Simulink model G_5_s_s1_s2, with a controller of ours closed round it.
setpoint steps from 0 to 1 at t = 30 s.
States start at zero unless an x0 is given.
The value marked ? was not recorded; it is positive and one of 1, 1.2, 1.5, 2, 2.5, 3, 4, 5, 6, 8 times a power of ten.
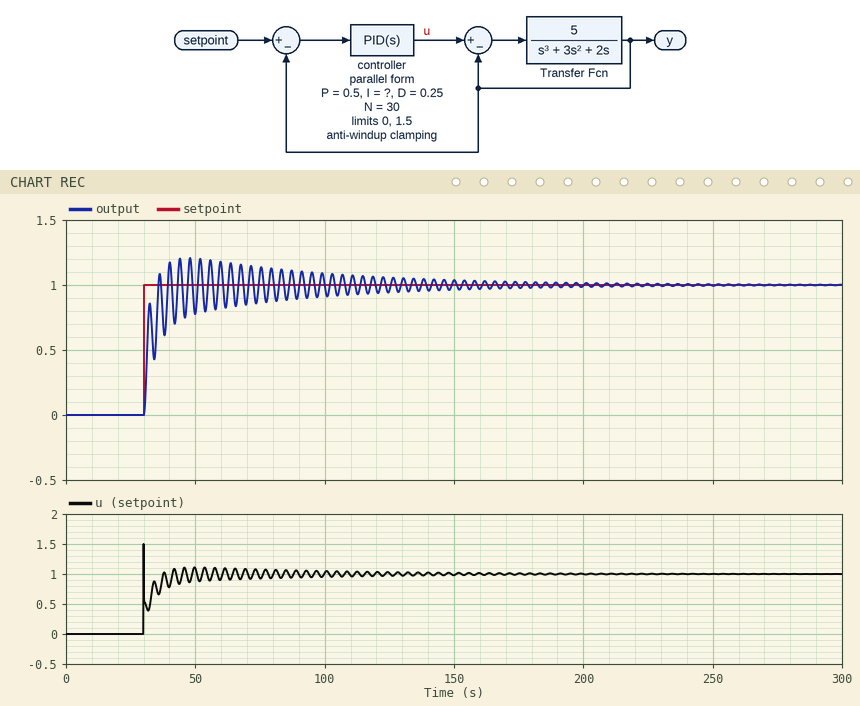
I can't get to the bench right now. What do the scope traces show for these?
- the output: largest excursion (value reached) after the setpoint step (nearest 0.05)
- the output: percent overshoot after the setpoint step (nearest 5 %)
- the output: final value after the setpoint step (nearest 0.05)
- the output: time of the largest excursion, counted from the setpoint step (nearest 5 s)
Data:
1.20
20 %
1.00
20 s
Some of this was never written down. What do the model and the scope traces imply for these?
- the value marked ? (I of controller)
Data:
0.3
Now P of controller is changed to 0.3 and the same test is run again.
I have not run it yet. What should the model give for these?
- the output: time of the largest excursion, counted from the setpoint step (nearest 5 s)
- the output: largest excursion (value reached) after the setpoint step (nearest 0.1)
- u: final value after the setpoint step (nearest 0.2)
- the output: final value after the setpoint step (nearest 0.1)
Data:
15 s
1.1
1.0
1.0
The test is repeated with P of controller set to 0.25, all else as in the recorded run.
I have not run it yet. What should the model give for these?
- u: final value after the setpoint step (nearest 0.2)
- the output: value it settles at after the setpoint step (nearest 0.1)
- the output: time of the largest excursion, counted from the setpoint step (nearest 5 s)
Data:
1.0
1.0
15 s
